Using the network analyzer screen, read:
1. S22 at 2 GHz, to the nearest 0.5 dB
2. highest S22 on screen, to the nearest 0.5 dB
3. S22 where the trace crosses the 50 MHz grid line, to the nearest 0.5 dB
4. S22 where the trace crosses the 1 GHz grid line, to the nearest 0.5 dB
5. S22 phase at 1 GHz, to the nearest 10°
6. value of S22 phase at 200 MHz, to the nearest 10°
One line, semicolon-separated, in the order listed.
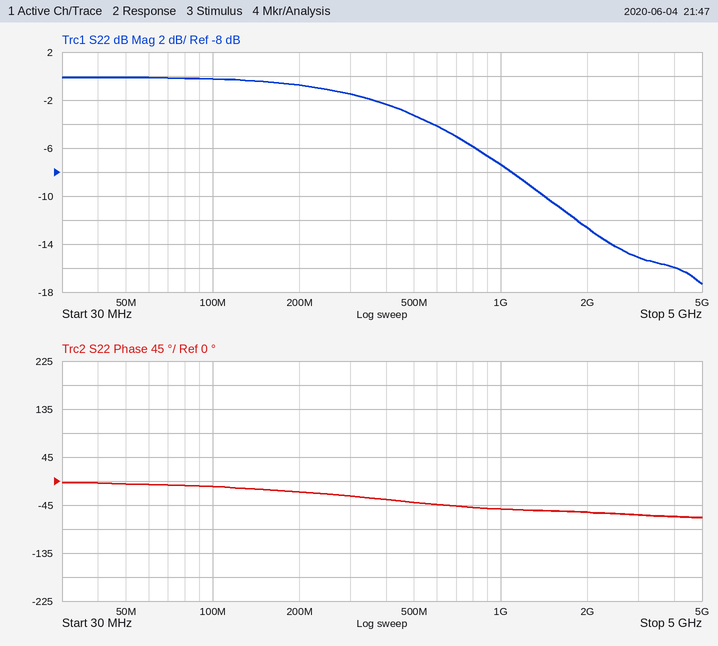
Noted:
-12.5 dB; 0.0 dB; 0.0 dB; -7.5 dB; -50°; -20°
